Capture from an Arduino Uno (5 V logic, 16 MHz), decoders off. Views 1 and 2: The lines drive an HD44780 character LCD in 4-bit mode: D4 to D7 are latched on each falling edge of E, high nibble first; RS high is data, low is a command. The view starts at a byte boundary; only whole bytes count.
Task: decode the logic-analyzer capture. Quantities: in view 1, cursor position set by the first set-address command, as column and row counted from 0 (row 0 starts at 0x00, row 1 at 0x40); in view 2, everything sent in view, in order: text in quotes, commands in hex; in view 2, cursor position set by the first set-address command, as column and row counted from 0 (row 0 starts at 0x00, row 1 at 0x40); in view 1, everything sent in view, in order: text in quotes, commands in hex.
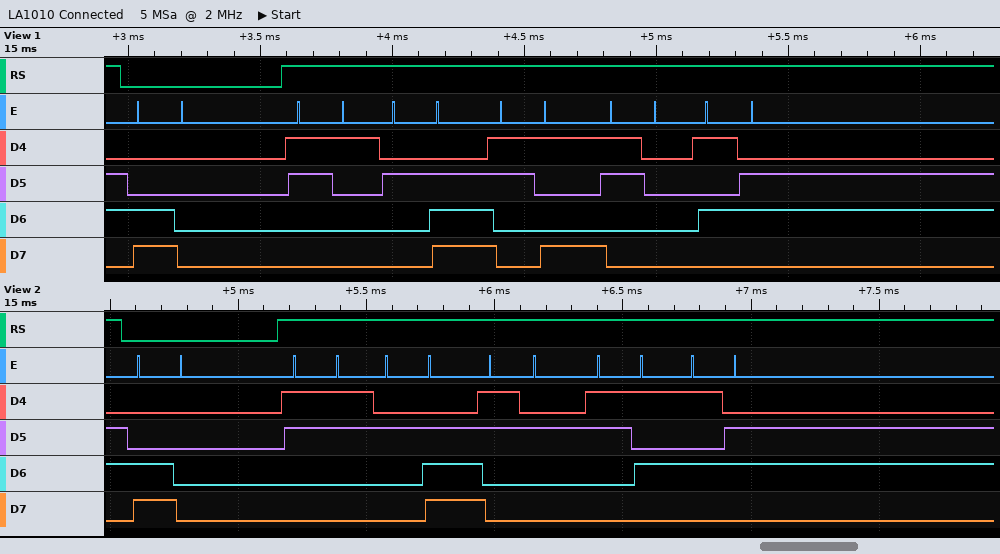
column 0, row 1
0xC0 "3.25V"
column 0, row 1
0xC0 "1.90V"
